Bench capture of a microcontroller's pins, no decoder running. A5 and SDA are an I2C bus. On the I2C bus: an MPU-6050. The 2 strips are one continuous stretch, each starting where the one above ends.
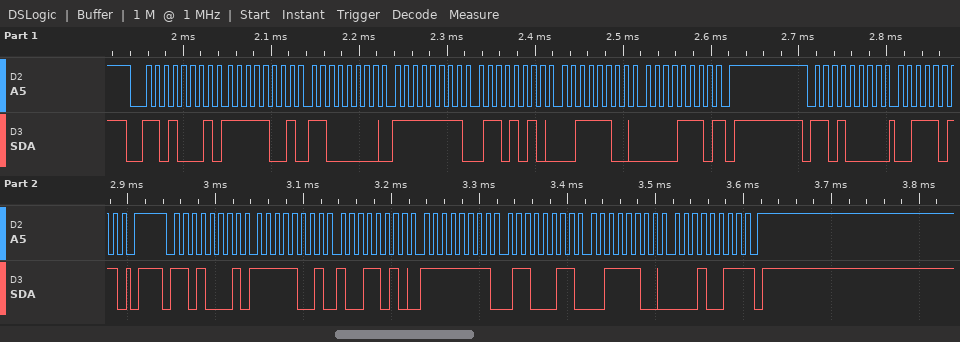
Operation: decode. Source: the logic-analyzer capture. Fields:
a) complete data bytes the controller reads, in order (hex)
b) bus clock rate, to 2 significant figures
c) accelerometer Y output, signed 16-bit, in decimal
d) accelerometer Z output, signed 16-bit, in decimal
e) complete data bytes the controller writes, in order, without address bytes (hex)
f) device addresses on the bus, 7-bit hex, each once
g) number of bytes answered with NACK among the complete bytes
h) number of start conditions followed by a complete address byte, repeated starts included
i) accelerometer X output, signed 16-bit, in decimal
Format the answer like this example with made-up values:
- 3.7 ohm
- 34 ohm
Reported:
- F9 C0 FF 6A 3C 0E F9 9A FF 63 3C 13
- 100 kHz
- -157
- 15379
- 3B
- 0x68
- 2
- 3
- -1638
